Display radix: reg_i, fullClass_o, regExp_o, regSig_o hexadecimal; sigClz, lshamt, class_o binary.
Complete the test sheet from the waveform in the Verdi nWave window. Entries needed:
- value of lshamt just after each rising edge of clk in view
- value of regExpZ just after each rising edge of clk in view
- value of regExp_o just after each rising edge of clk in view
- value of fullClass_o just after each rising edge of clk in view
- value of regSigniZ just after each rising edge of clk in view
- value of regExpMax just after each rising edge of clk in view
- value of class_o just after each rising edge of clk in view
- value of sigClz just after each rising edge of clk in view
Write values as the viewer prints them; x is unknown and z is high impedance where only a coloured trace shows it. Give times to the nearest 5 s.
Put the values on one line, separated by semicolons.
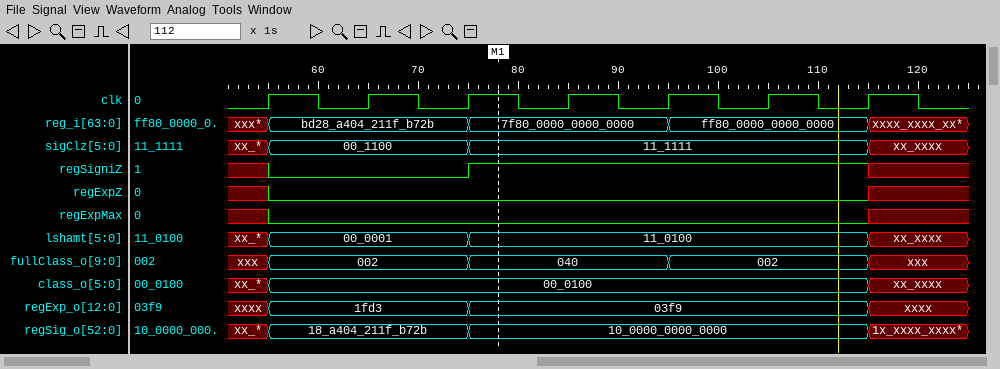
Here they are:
00_0001, 00_0001, 11_0100, 11_0100, 11_0100, 11_0100, xx_xxxx; 0 0 0 0 0 0 x; 1fd3, 1fd3, 03f9, 03f9, 03f9, 03f9, xxxx; 002, 002, 040, 040, 002, 002, xxx; 0 0 1 1 1 1 x; 0 0 0 0 0 0 x; 00_0100, 00_0100, 00_0100, 00_0100, 00_0100, 00_0100, xx_xxxx; 00_1100, 00_1100, 11_1111, 11_1111, 11_1111, 11_1111, xx_xxxx
